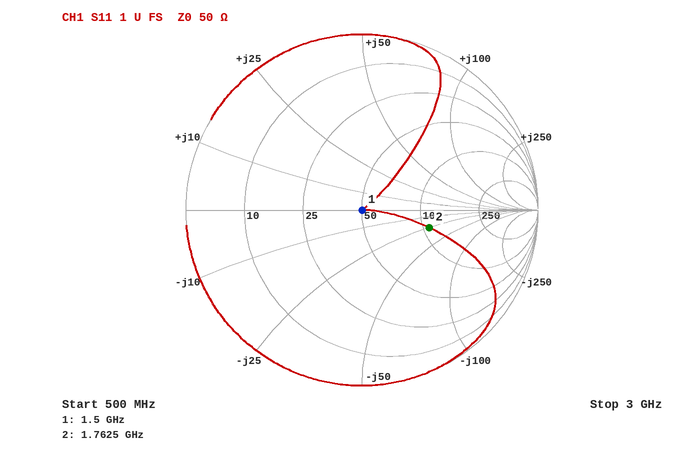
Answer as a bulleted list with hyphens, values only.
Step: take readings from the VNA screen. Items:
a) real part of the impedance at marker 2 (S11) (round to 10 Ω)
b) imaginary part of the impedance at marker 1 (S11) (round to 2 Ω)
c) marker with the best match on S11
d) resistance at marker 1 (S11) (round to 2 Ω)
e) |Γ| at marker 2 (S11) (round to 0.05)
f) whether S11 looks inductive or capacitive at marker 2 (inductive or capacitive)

- 110 Ω
- 0 Ω
- marker 1
- 50 Ω
- 0.40
- capacitive
